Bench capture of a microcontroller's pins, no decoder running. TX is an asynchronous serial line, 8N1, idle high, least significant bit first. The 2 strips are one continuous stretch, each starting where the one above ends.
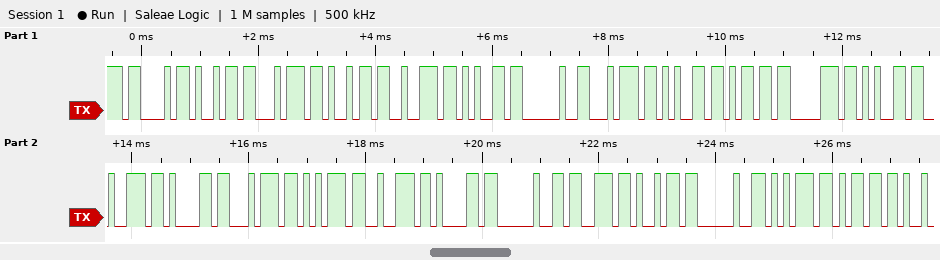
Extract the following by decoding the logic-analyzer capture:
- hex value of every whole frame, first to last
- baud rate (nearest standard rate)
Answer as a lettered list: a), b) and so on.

a) 43 69 74 69 72 65 20 74 65 6D 70 65 72 61 74 75 72 61 20 73 69 20 75 6D
b) 9600 baud
